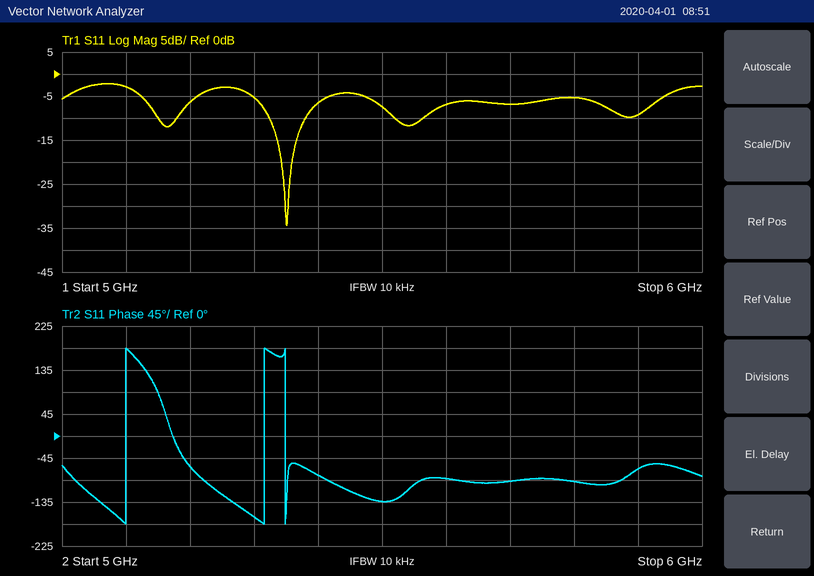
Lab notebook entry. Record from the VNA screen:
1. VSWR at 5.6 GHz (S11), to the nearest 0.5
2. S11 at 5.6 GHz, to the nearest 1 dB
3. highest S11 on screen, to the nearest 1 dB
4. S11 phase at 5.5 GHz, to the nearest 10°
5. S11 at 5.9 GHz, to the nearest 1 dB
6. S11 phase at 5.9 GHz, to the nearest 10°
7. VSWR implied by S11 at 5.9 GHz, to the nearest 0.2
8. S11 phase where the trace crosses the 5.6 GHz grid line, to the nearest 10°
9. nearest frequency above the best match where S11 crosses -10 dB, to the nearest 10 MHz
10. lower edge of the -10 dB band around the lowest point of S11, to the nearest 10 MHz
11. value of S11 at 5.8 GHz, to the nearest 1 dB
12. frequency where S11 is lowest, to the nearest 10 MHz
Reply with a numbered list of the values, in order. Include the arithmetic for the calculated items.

1. |Γ| = 10^(-7/20) = 0.4467; VSWR = (1 + 0.4467)/(1 − 0.4467) ≈ 2.61, so 2.5 to the nearest 0.5
2. -7 dB
3. -2 dB
4. -130°
5. -9 dB
6. -70°
7. |Γ| = 10^(-9/20) = 0.3548; VSWR = (1 + 0.3548)/(1 − 0.3548) ≈ 2.10, so 2.0 to the nearest 0.2
8. -90°
9. 5.38 GHz
10. 5.32 GHz
11. -5 dB
12. 5.35 GHz
